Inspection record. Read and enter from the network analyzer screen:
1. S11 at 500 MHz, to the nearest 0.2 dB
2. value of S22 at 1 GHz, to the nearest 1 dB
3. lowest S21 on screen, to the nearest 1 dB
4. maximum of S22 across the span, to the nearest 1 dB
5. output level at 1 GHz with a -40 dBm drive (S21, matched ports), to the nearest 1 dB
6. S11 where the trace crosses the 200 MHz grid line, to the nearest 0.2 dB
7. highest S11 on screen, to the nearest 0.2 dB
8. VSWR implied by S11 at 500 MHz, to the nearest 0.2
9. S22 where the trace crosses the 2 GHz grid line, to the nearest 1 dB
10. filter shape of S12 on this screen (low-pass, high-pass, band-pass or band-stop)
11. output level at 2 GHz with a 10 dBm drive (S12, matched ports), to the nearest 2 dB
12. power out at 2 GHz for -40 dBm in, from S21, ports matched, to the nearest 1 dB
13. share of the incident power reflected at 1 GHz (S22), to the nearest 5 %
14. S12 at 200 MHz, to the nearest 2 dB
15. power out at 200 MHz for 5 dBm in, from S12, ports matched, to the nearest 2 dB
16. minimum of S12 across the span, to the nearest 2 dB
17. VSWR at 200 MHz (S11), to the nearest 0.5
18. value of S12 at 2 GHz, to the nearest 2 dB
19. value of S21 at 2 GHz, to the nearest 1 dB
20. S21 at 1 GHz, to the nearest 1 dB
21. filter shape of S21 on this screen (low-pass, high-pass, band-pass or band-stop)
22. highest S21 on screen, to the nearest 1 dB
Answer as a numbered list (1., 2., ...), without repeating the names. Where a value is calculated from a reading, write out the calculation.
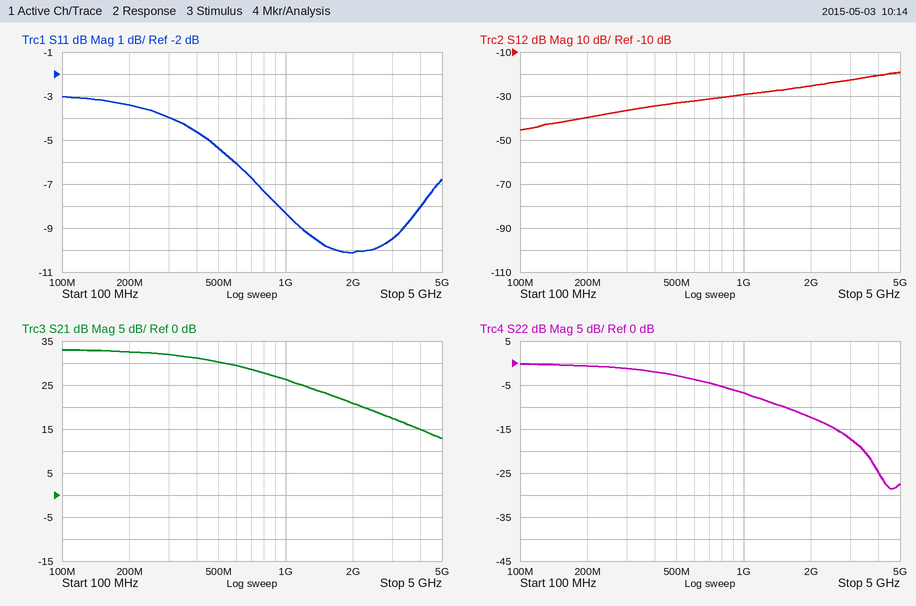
1. -5.4 dB
2. -7 dB
3. 13 dB
4. 0 dB
5. -40 dBm + (26 dB) = -14 dBm
6. -3.4 dB
7. -3.0 dB
8. |Γ| = 10^(-5.4/20) = 0.5370; VSWR = (1 + 0.5370)/(1 − 0.5370) ≈ 3.32, so 3.4 to the nearest 0.2
9. -12 dB
10. high-pass
11. 10 dBm + (-26 dB) = -16 dBm
12. -40 dBm + (21 dB) = -19 dBm
13. 10^(-7/10) ≈ 20 %
14. -40 dB
15. 5 dBm + (-40 dB) = -34 dBm
16. -46 dB
17. |Γ| = 10^(-3.4/20) = 0.6761; VSWR = (1 + 0.6761)/(1 − 0.6761) ≈ 5.17, so 5.0 to the nearest 0.5
18. -26 dB
19. 21 dB
20. 26 dB
21. low-pass
22. 33 dB
